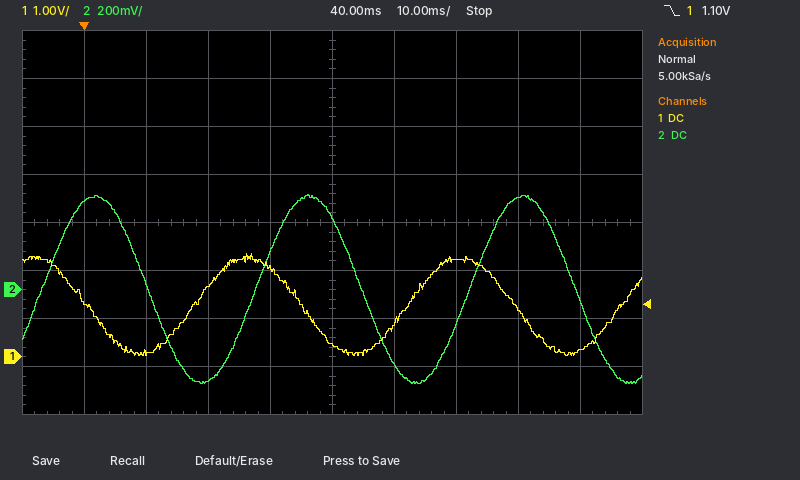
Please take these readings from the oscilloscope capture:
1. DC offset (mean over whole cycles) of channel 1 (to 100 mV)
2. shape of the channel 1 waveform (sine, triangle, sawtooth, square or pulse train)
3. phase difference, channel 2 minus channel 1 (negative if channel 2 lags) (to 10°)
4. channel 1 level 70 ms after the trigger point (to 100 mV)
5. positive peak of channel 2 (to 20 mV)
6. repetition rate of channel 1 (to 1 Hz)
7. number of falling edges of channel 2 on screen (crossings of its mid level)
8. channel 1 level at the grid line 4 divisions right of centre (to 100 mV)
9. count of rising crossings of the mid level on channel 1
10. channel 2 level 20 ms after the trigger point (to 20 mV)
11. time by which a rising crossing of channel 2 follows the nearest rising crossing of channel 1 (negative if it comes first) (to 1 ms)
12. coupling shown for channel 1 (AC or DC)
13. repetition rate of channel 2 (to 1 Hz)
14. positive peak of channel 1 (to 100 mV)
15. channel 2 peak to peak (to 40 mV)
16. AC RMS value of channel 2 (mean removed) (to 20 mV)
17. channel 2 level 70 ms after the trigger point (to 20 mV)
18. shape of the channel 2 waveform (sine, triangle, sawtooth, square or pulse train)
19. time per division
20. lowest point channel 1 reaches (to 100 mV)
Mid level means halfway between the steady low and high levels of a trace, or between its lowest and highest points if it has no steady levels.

1.1 V
sine
-100°
1.0 V
400 mV
29 Hz
3
100 mV
3
-380 mV
+10 ms
DC
29 Hz
2.2 V
800 mV
280 mV
380 mV
sine
10 ms
0.0 V
